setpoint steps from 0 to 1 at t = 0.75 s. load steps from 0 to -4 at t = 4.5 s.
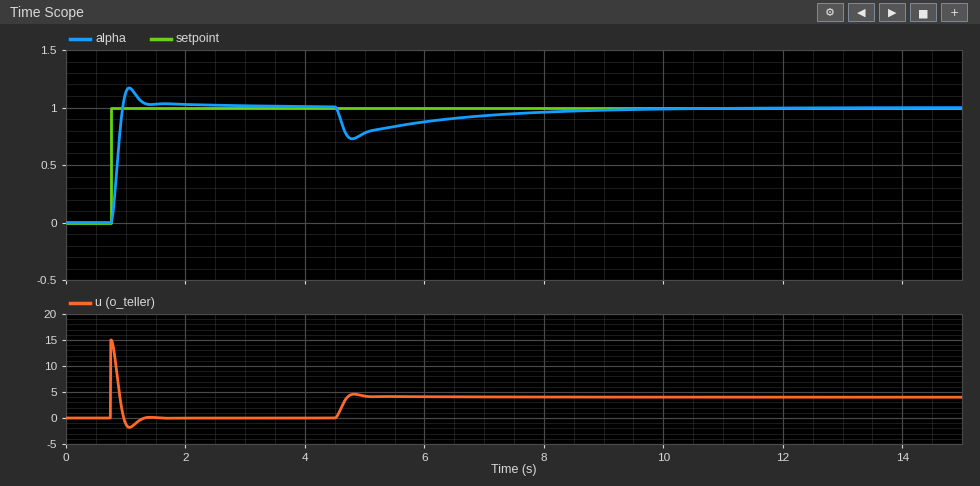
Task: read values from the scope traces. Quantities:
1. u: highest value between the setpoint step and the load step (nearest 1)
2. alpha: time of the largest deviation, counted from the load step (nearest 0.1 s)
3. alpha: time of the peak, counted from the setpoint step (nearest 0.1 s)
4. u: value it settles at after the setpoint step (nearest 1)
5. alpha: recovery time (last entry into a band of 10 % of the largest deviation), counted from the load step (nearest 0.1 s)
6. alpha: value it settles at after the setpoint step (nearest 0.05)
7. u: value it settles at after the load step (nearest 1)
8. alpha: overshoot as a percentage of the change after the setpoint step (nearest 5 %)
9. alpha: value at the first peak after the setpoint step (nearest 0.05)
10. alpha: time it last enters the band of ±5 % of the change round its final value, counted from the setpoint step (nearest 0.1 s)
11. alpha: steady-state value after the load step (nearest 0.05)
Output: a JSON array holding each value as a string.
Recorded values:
["15", "0.3 s", "0.3 s", "0", "4.2 s", "1.00", "4", "15 %", "1.15", "0.5 s", "1.00"]
